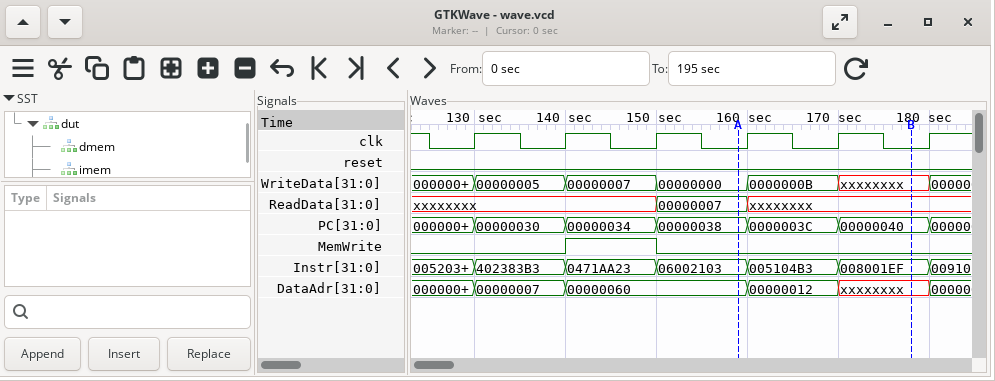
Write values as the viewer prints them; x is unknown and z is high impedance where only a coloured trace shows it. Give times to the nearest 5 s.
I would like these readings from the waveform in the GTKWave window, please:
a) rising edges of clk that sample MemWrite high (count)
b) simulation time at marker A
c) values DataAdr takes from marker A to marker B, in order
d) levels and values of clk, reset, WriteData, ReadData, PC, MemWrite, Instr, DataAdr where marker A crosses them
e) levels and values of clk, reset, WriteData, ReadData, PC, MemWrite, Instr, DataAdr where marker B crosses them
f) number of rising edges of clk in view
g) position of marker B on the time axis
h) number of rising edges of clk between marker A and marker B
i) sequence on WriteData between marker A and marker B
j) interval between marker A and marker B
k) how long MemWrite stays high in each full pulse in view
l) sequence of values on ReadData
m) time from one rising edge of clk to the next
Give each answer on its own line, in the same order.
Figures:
1
160 s
00000060, 00000012, xxxxxxxx
clk=0, reset=0, WriteData=00000000, ReadData=00000007, PC=00000038, MemWrite=0, Instr=06002103, DataAdr=00000060
clk=0, reset=0, WriteData=xxxxxxxx, ReadData=xxxxxxxx, PC=00000040, MemWrite=0, Instr=008001EF, DataAdr=xxxxxxxx
6
180 s
2
00000000, 0000000B, xxxxxxxx
20 s
10 s
xxxxxxxx, 00000007, xxxxxxxx
10 s
